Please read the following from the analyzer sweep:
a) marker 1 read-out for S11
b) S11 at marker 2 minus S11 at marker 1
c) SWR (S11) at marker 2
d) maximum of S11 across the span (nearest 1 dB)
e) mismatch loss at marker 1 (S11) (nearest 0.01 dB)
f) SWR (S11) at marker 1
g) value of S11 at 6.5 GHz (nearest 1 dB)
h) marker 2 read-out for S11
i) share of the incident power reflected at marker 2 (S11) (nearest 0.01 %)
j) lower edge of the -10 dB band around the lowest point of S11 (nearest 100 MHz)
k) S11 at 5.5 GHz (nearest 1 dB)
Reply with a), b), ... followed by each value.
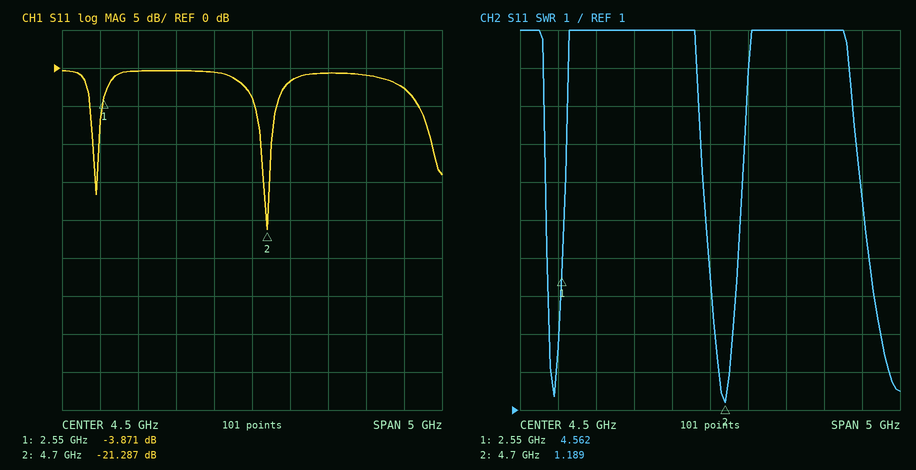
a) -3.871 dB
b) -17.416 dB
c) 1.189
d) 0 dB
e) 2.29 dB
f) 4.562
g) -3 dB
h) -21.287 dB
i) 0.74 %
j) 4.6 GHz
k) -1 dB
